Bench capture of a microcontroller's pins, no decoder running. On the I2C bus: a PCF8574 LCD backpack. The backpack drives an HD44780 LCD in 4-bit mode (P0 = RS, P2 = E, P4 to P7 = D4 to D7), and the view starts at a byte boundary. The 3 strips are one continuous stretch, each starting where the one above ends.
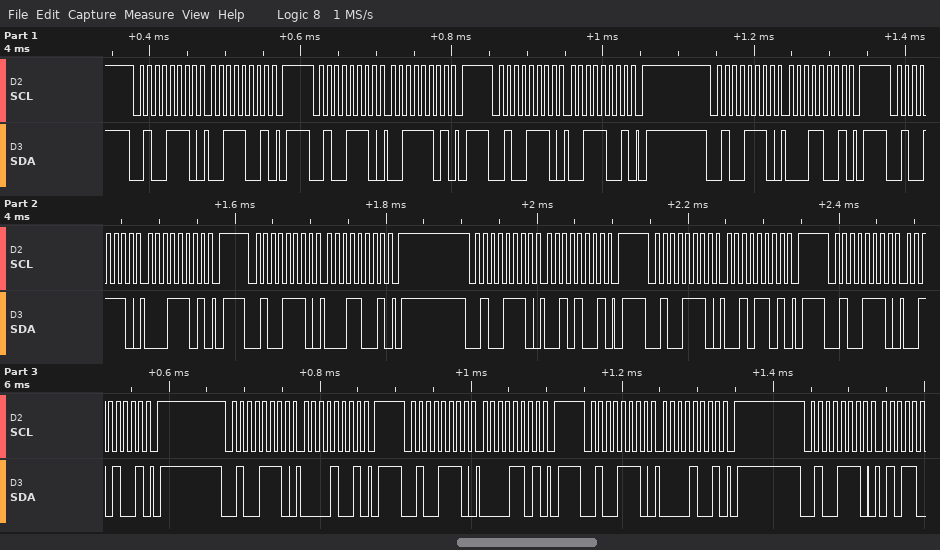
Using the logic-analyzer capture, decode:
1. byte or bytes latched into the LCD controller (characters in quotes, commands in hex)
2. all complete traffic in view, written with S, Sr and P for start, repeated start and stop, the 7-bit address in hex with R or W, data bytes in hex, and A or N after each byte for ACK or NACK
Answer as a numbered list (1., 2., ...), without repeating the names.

1. '1' ' '
2. S 27W A 39 A P S 27W A 3D A P S 27W A 39 A P S 27W A 19 A P S 27W A 1D A P S 27W A 19 A P S 27W A 29 A P S 27W A 2D A P S 27W A 29 A P S 27W A 09 A P S 27W A 0D A P S 27W A 09 A P S 27W A
